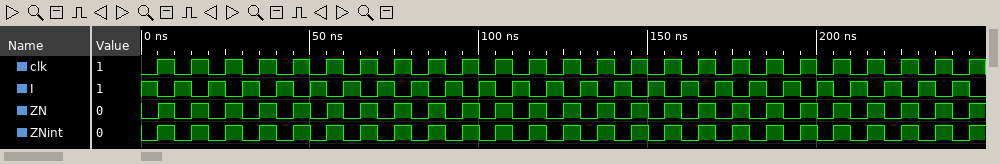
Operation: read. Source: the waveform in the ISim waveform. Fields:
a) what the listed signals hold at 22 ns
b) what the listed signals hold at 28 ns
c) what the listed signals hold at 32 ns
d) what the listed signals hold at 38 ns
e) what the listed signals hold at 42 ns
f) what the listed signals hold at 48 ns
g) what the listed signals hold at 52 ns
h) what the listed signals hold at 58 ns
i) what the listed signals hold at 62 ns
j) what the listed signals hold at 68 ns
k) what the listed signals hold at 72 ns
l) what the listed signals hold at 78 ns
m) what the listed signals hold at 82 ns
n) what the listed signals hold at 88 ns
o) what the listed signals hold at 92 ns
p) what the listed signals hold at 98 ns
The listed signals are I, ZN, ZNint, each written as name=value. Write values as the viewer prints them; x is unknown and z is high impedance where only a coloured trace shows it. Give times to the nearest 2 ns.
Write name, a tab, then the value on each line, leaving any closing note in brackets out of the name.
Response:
what the listed signals hold at 22 ns	I=1, ZN=0, ZNint=0
what the listed signals hold at 28 ns	I=0, ZN=1, ZNint=1
what the listed signals hold at 32 ns	I=1, ZN=0, ZNint=0
what the listed signals hold at 38 ns	I=0, ZN=1, ZNint=1
what the listed signals hold at 42 ns	I=1, ZN=0, ZNint=0
what the listed signals hold at 48 ns	I=0, ZN=1, ZNint=1
what the listed signals hold at 52 ns	I=1, ZN=0, ZNint=0
what the listed signals hold at 58 ns	I=0, ZN=1, ZNint=1
what the listed signals hold at 62 ns	I=1, ZN=0, ZNint=0
what the listed signals hold at 68 ns	I=0, ZN=1, ZNint=1
what the listed signals hold at 72 ns	I=1, ZN=0, ZNint=0
what the listed signals hold at 78 ns	I=0, ZN=1, ZNint=1
what the listed signals hold at 82 ns	I=1, ZN=0, ZNint=0
what the listed signals hold at 88 ns	I=0, ZN=1, ZNint=1
what the listed signals hold at 92 ns	I=1, ZN=0, ZNint=0
what the listed signals hold at 98 ns	I=0, ZN=1, ZNint=1
